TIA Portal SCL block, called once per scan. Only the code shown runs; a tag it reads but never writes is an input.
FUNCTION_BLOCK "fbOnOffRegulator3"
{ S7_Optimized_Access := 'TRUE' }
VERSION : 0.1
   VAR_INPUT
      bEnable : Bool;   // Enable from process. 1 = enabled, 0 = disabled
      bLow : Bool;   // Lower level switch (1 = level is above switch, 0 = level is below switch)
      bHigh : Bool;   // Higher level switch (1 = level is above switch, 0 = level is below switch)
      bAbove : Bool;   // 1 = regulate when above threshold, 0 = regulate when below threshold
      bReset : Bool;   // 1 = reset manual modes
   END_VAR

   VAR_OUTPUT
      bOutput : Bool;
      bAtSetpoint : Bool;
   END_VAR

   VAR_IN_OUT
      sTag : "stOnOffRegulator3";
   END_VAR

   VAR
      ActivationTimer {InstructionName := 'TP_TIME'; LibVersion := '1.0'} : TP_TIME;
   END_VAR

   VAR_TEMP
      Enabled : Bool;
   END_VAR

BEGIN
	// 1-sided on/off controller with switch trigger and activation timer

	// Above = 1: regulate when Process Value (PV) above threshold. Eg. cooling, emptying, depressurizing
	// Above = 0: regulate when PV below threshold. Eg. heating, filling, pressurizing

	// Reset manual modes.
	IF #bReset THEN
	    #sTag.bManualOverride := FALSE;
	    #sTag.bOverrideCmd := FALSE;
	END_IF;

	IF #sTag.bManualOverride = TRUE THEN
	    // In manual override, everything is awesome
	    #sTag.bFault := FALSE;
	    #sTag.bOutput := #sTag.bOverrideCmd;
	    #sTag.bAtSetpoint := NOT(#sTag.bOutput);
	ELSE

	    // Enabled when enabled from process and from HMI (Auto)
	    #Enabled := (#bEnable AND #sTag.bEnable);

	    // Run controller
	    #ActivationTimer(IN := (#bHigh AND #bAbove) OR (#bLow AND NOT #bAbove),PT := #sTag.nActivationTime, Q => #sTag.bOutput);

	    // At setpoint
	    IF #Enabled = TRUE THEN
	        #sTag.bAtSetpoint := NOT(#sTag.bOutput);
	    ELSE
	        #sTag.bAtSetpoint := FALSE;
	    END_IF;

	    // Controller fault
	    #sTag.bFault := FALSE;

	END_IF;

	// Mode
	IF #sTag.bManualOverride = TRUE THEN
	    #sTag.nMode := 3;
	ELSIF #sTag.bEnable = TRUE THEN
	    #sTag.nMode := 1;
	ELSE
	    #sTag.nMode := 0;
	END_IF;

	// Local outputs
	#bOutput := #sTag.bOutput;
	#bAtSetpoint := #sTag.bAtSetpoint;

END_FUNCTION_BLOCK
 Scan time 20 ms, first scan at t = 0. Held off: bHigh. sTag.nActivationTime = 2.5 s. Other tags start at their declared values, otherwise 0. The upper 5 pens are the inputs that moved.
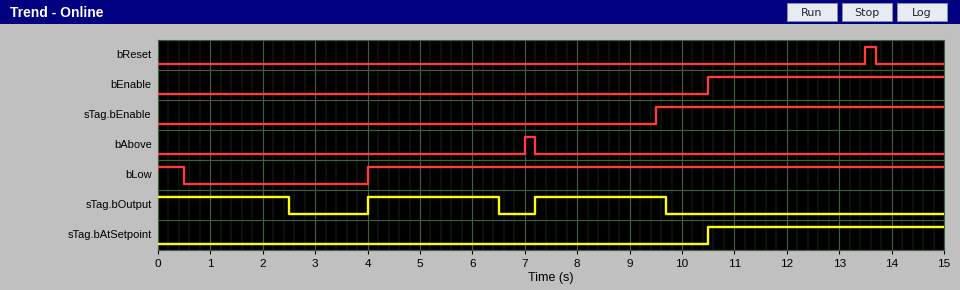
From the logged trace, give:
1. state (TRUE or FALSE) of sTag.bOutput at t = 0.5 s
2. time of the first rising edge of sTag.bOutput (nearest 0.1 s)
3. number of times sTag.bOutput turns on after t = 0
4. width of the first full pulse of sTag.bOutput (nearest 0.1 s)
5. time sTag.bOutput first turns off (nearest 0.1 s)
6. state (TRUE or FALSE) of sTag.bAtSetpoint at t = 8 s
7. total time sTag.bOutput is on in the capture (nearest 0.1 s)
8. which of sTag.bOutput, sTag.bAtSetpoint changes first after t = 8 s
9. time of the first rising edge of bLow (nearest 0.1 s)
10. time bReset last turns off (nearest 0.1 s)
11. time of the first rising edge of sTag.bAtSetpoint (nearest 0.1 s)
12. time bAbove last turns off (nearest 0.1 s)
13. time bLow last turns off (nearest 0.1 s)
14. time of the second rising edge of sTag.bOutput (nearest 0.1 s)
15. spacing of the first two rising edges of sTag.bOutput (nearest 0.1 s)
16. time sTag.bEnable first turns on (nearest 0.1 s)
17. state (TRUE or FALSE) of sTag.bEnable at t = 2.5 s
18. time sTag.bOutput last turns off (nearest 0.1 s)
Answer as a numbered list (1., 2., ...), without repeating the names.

1. TRUE
2. 4.0 s
3. 2
4. 2.5 s
5. 2.5 s
6. FALSE
7. 7.5 s
8. sTag.bOutput
9. 4.0 s
10. 13.7 s
11. 10.5 s
12. 7.2 s
13. 0.5 s
14. 7.2 s
15. 3.2 s
16. 9.5 s
17. FALSE
18. 9.7 s
